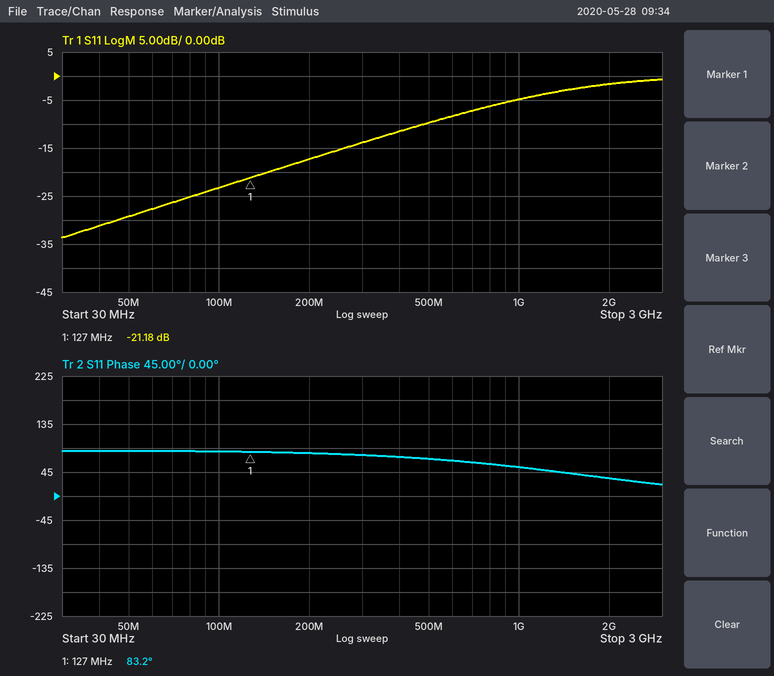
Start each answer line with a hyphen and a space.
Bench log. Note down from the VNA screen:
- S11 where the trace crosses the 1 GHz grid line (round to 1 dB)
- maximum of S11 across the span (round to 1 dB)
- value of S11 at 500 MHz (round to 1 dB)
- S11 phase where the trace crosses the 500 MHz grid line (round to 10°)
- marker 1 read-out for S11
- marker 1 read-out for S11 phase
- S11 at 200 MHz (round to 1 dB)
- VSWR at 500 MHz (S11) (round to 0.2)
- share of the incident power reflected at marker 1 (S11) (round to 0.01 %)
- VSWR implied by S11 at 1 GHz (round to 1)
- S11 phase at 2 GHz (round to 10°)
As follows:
- -5 dB
- -1 dB
- -10 dB
- 70°
- -21.18 dB
- 83.2°
- -17 dB
- 2.0
- 0.76 %
- 4
- 30°
